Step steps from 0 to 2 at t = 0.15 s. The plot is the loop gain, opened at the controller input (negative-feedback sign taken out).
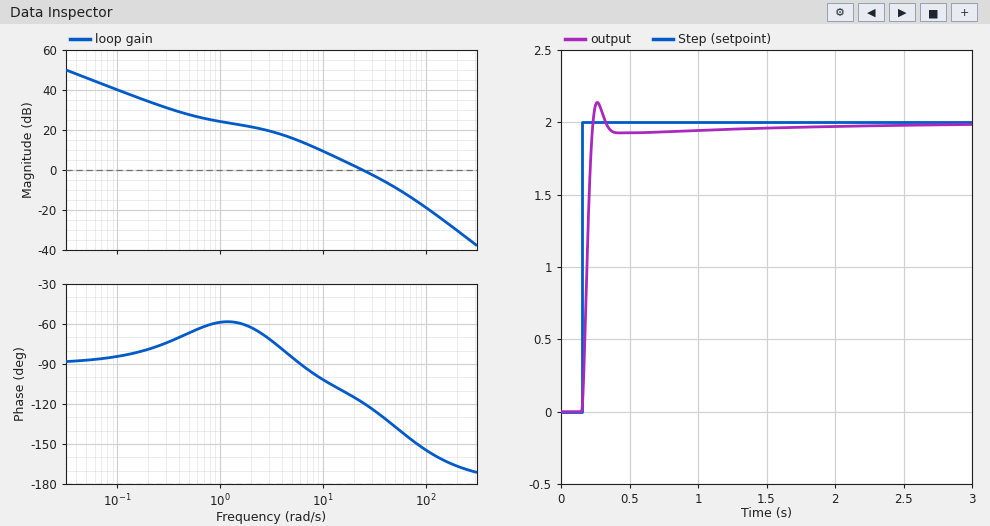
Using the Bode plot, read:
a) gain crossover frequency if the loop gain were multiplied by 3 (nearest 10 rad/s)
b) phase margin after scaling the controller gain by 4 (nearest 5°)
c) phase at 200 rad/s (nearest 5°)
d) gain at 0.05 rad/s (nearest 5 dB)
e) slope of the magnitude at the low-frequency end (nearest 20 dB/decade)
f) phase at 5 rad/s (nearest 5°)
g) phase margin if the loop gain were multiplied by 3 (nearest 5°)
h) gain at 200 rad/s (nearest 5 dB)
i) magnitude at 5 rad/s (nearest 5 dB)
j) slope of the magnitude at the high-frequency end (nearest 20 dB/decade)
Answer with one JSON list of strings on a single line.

["50 rad/s", "35°", "-165°", "45 dB", "-20 dB/decade", "-85°", "40°", "-30 dB", "15 dB", "-40 dB/decade"]
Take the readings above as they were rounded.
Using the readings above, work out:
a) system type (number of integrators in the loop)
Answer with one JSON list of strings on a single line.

["1"]
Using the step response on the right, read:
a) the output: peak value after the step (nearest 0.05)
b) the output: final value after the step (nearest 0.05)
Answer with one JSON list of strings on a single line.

["2.15", "2.00"]
